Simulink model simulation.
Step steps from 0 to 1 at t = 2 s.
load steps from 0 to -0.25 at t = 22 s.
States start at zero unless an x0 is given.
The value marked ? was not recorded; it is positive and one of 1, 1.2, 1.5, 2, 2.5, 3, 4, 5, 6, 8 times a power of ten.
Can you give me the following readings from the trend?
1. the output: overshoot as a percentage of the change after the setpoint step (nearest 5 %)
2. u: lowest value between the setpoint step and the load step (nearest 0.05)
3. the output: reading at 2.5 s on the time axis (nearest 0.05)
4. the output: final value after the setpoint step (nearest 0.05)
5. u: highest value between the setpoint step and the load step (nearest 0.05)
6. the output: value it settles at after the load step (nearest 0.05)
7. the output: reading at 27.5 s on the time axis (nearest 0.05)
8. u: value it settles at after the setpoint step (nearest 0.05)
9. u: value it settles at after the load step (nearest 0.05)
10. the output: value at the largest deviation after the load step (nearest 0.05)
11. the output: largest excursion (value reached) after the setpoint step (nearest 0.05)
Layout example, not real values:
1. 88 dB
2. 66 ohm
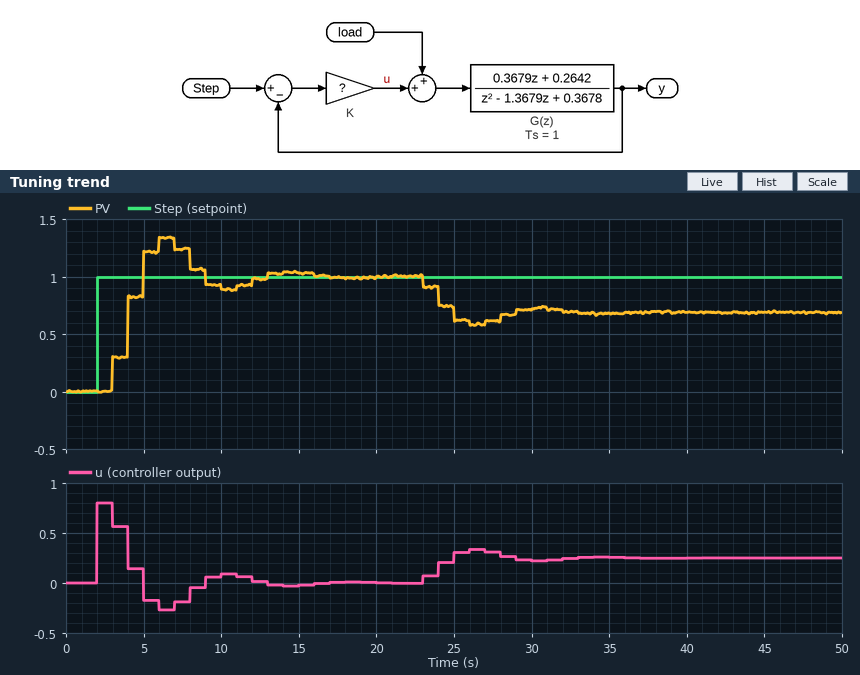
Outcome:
1. 35 %
2. -0.25
3. 0.00
4. 1.00
5. 0.80
6. 0.70
7. 0.60
8. 0.00
9. 0.25
10. 0.60
11. 1.35
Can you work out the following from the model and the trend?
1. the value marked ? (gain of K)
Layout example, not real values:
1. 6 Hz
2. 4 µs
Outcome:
1. 0.8
